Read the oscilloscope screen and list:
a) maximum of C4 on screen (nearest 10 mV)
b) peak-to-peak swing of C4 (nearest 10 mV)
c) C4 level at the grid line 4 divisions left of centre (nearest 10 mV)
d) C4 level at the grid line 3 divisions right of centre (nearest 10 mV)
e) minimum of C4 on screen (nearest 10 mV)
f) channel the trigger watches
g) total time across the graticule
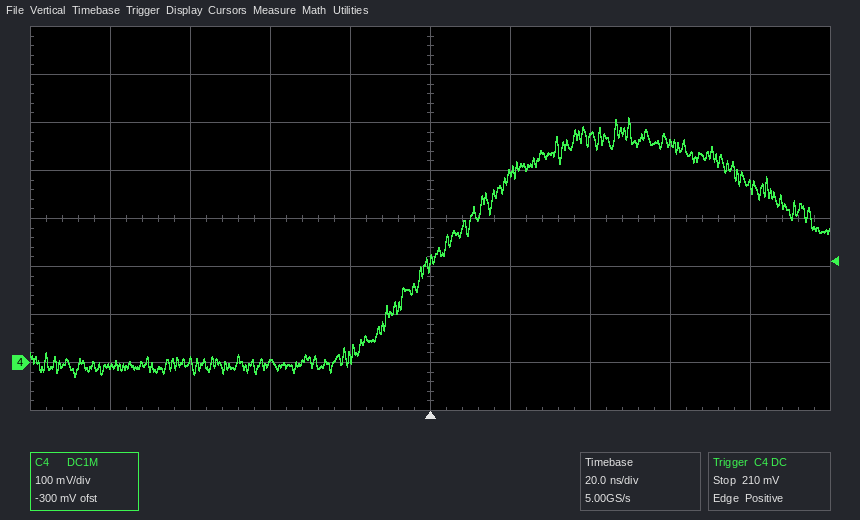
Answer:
510 mV
540 mV
-10 mV
460 mV
-30 mV
C4
200 ns
